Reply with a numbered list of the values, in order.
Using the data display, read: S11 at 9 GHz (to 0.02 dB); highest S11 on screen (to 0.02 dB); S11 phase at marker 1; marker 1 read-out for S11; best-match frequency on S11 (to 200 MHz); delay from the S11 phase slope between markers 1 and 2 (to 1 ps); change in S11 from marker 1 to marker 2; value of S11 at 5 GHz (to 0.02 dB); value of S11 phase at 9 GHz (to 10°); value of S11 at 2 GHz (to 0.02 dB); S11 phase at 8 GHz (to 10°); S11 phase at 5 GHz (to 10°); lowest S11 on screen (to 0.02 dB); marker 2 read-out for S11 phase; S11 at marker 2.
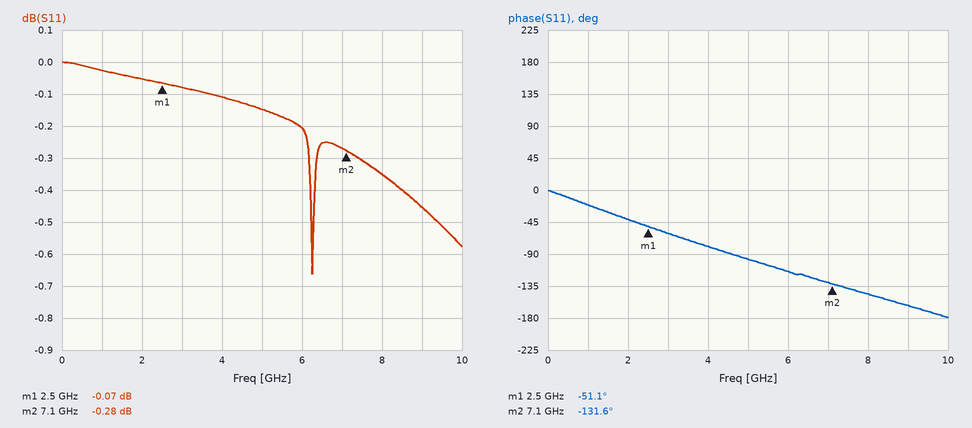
1. -0.46 dB
2. 0.00 dB
3. -51.1°
4. -0.07 dB
5. 6.2 GHz
6. 49 ps
7. -0.21 dB
8. -0.14 dB
9. -160°
10. -0.06 dB
11. -150°
12. -100°
13. -0.66 dB
14. -131.6°
15. -0.28 dB
